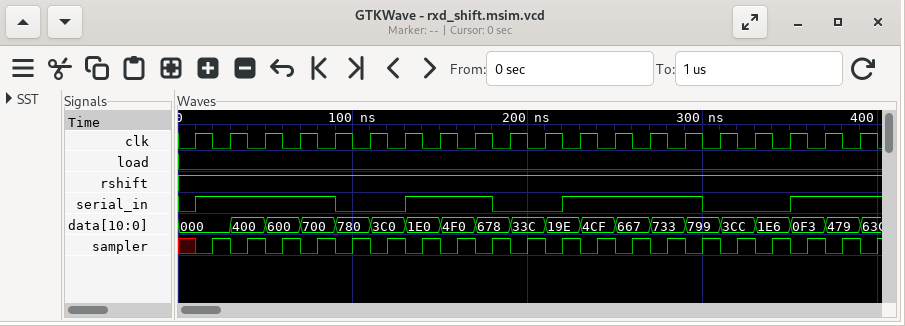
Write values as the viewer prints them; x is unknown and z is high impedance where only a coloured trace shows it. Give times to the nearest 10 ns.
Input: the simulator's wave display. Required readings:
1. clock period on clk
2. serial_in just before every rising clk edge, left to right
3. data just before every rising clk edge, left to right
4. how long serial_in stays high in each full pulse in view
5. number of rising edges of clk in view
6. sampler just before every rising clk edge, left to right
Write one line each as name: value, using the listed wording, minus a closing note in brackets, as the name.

clock period on clk: 20 ns
serial_in just before every rising clk edge, left to right: 0 1 1 1 1 0 0 1 1 0 0 1 1 1 1 0 0 0 1 1
data just before every rising clk edge, left to right: 000, 000, 400, 600, 700, 780, 3C0, 1E0, 4F0, 678, 33C, 19E, 4CF, 667, 733, 799, 3CC, 1E6, 0F3, 479
how long serial_in stays high in each full pulse in view: 80 ns, 50 ns, 80 ns
number of rising edges of clk in view: 20
sampler just before every rising clk edge, left to right: x 1 1 1 1 1 1 1 1 1 1 1 1 1 1 1 1 1 1 1
